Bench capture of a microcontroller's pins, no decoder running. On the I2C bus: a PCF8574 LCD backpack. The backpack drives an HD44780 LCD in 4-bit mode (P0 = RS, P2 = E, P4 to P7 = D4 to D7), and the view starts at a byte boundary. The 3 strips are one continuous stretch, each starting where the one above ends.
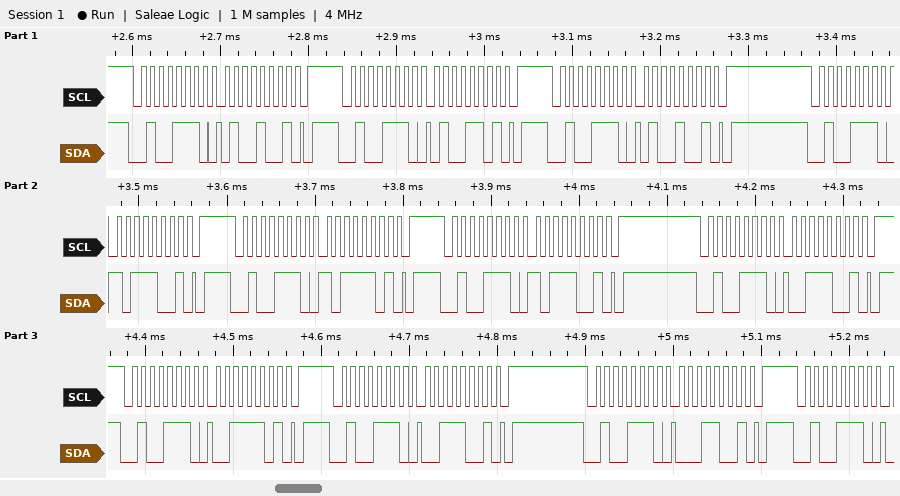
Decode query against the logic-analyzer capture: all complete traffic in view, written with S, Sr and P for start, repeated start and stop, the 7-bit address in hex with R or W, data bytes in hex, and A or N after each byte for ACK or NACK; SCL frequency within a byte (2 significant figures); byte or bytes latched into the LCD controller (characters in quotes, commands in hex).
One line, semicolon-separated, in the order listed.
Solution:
S 27W A 49 A P S 27W A 4D A P S 27W A 49 A P S 27W A B9 A P S 27W A BD A P S 27W A B9 A P S 27W A 39 A P S 27W A 3D A P S 27W A 39 A P S 27W A 19 A P S 27W A; 100 kHz; 'K'
